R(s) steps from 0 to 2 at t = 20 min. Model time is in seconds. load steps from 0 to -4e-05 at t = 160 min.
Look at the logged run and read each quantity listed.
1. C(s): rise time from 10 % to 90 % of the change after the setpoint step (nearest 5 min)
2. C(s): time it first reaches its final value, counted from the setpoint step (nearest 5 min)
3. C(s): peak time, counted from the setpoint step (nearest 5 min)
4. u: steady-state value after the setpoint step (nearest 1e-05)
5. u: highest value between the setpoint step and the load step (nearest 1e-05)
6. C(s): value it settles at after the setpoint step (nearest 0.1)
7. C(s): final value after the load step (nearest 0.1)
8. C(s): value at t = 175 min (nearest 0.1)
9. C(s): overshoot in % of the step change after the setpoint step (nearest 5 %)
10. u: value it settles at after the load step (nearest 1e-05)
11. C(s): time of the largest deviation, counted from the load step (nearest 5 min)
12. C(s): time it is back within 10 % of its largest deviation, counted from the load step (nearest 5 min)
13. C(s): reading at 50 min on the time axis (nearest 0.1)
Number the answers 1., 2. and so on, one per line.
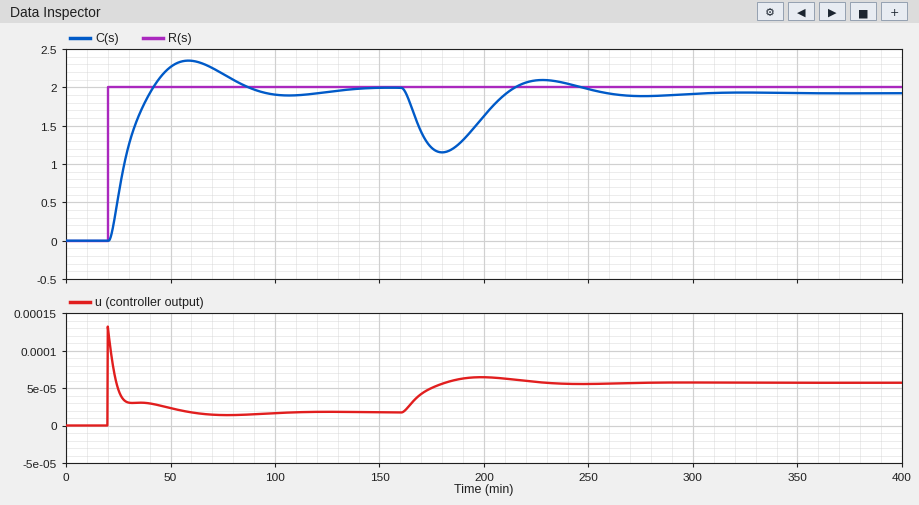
1. 15 min
2. 20 min
3. 40 min
4. 0.00002
5. 0.00013
6. 2.0
7. 1.9
8. 1.2
9. 20 %
10. 0.00006
11. 20 min
12. 85 min
13. 2.3
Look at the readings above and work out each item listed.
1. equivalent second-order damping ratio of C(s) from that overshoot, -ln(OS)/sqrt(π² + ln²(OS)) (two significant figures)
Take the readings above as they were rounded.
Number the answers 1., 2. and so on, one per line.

1. 0.46
